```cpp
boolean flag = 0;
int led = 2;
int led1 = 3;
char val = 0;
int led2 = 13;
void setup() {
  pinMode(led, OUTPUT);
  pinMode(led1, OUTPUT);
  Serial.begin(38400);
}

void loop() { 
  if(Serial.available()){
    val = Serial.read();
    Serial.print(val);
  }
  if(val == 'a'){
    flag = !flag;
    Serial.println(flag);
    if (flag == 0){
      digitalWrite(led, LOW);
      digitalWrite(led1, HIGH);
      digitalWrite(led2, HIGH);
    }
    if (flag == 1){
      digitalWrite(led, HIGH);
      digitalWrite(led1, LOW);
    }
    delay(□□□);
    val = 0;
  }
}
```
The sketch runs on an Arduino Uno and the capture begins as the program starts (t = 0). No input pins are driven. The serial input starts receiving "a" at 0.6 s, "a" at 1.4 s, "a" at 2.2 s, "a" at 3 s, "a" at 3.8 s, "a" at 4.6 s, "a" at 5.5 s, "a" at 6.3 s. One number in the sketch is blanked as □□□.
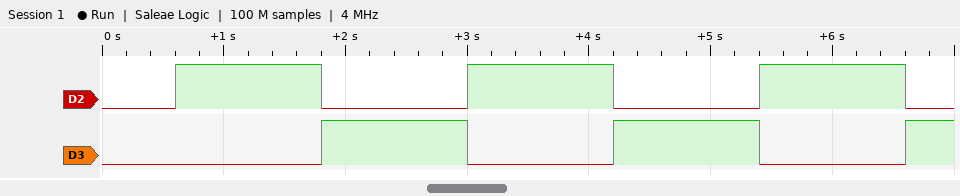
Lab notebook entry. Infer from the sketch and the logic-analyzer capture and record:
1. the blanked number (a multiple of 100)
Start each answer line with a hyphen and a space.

- 1200
